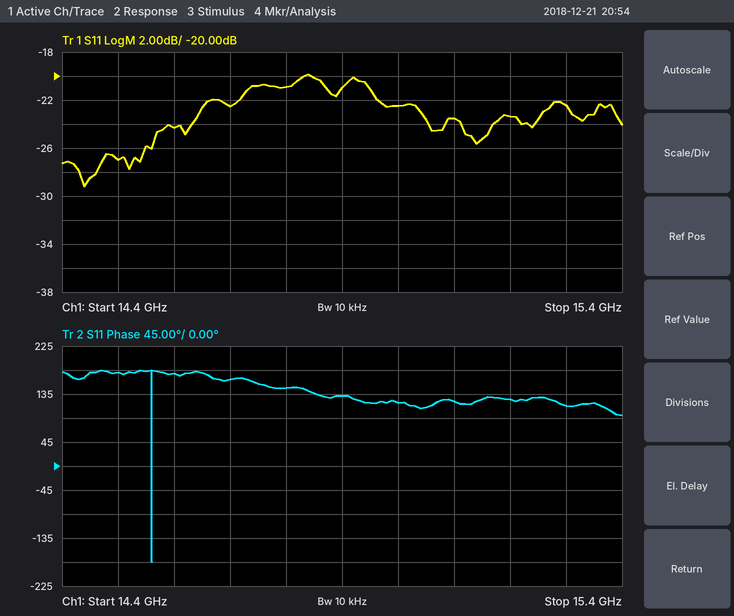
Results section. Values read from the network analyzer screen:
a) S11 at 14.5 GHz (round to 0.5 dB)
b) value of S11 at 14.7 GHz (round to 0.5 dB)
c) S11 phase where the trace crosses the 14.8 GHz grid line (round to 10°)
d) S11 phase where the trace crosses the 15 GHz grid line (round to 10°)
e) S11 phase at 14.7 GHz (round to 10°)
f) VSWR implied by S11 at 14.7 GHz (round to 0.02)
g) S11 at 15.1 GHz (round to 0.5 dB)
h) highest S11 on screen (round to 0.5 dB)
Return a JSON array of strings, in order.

["-27.0 dB", "-22.5 dB", "150°", "120°", "160°", "1.16", "-23.5 dB", "-20.0 dB"]
